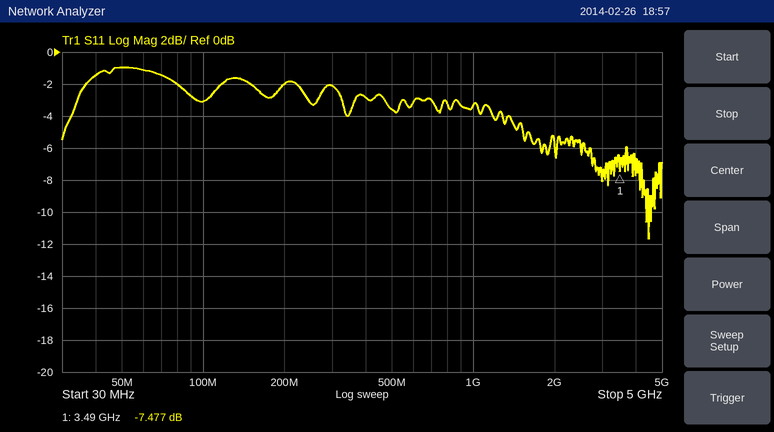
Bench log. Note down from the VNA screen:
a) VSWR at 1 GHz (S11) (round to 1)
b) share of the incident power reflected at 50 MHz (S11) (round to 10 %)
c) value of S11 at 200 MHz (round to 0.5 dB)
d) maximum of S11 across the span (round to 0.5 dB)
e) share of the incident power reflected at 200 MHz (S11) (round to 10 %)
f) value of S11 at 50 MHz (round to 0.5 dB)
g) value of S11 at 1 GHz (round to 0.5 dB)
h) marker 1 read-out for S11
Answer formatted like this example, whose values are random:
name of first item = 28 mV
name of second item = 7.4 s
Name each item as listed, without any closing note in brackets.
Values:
VSWR at 1 GHz (S11) = 5
share of the incident power reflected at 50 MHz (S11) = 80 %
value of S11 at 200 MHz = -2.0 dB
maximum of S11 across the span = -1.0 dB
share of the incident power reflected at 200 MHz (S11) = 60 %
value of S11 at 50 MHz = -1.0 dB
value of S11 at 1 GHz = -3.5 dB
marker 1 read-out for S11 = -7.477 dB
